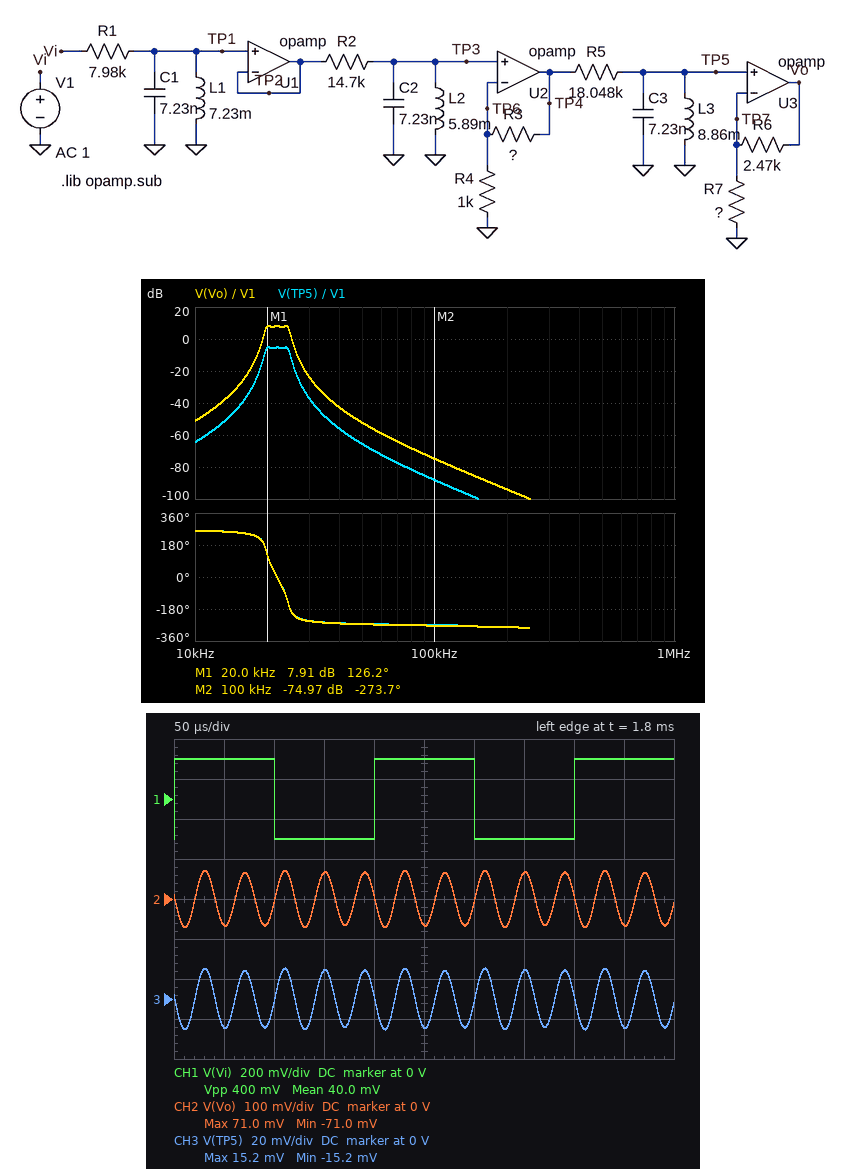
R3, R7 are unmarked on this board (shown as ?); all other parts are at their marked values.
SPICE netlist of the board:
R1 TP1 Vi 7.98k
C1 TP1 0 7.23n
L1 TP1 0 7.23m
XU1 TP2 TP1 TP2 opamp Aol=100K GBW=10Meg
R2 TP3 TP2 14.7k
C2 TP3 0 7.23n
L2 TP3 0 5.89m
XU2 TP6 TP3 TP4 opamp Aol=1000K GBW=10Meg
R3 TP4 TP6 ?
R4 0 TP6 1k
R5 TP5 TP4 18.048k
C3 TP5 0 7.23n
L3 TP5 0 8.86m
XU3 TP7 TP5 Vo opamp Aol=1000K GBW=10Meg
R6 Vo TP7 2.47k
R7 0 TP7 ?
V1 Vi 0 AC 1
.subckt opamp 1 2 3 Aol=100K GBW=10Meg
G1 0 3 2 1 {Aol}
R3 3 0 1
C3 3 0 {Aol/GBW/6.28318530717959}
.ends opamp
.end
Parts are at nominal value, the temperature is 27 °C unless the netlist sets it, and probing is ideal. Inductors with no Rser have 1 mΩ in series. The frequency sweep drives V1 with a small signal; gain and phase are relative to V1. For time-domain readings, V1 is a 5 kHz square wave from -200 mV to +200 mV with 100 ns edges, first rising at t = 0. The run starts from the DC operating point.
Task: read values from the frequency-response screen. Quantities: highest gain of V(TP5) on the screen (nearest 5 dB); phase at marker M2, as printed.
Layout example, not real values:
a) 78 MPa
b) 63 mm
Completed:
a) -5 dB
b) -273.7 deg
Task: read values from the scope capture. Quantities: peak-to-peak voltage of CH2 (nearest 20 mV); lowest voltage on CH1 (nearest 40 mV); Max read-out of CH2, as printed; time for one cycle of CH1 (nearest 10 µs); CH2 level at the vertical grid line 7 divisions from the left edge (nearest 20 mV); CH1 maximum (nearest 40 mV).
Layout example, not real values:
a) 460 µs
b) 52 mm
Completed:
a) 140 mV
b) -200 mV
c) 71.0 mV
d) 200 µs
e) 60 mV
f) 200 mV
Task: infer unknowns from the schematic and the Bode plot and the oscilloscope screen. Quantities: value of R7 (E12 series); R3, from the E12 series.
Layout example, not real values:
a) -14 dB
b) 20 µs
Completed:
a) 680 Ω
b) 5.6 kΩ
